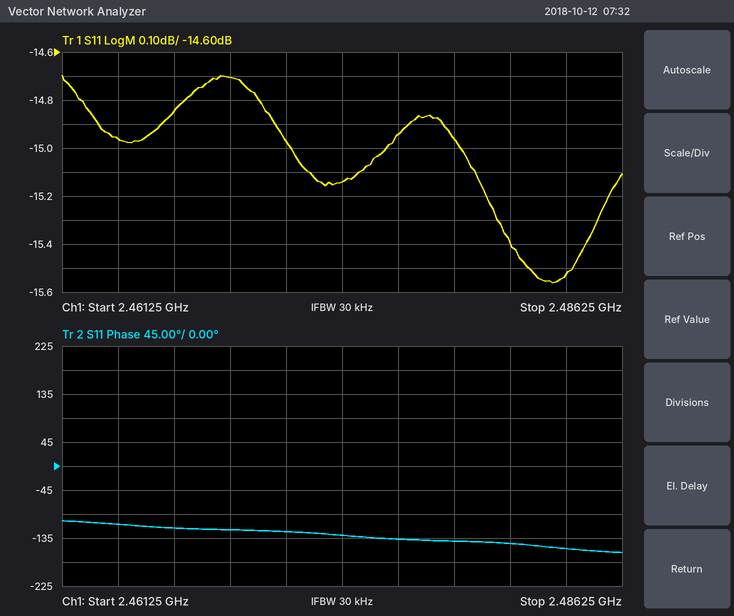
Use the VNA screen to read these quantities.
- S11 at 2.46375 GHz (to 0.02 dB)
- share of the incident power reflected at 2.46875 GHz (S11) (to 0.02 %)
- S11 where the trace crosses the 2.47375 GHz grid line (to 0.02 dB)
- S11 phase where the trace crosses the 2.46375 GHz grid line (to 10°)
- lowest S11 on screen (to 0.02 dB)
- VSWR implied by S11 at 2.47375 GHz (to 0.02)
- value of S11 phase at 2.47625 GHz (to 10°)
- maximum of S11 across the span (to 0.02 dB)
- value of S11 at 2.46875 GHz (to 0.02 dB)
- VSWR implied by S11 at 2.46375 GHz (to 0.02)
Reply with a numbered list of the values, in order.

1. -14.96 dB
2. 3.38 %
3. -15.14 dB
4. -110°
5. -15.56 dB
6. 1.42
7. -140°
8. -14.70 dB
9. -14.70 dB
10. 1.44
